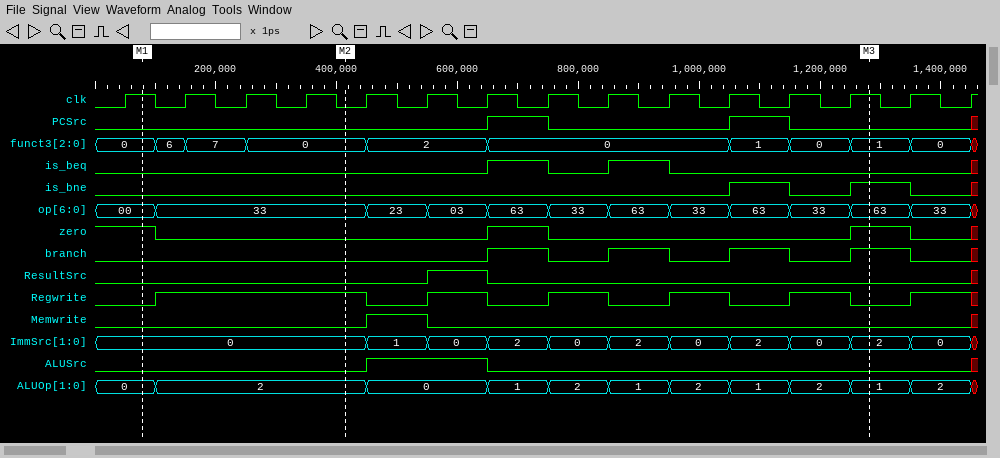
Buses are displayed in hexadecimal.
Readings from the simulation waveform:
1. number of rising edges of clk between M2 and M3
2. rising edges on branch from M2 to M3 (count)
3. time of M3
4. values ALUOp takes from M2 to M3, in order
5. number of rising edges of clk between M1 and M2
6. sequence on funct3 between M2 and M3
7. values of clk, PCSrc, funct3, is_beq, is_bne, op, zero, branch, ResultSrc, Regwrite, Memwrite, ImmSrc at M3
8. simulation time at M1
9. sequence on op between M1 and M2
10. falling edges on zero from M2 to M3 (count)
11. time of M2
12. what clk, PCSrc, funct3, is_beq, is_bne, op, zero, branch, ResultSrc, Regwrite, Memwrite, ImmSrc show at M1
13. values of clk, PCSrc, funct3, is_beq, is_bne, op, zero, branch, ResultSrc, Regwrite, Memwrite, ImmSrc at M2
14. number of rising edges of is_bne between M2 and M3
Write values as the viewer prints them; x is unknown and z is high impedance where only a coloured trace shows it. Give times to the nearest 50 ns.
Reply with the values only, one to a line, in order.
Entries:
9
4
1300 ns
2, 0, 1, 2, 1, 2, 1, 2, 1
3
0, 2, 0, 1, 0, 1
clk=1, PCSrc=0, funct3=1, is_beq=0, is_bne=1, op=63, zero=1, branch=1, ResultSrc=0, Regwrite=0, Memwrite=0, ImmSrc=2
100 ns
00, 33
1
400 ns
clk=1, PCSrc=0, funct3=0, is_beq=0, is_bne=0, op=00, zero=1, branch=0, ResultSrc=0, Regwrite=0, Memwrite=0, ImmSrc=0
clk=0, PCSrc=0, funct3=0, is_beq=0, is_bne=0, op=33, zero=0, branch=0, ResultSrc=0, Regwrite=1, Memwrite=0, ImmSrc=0
2
